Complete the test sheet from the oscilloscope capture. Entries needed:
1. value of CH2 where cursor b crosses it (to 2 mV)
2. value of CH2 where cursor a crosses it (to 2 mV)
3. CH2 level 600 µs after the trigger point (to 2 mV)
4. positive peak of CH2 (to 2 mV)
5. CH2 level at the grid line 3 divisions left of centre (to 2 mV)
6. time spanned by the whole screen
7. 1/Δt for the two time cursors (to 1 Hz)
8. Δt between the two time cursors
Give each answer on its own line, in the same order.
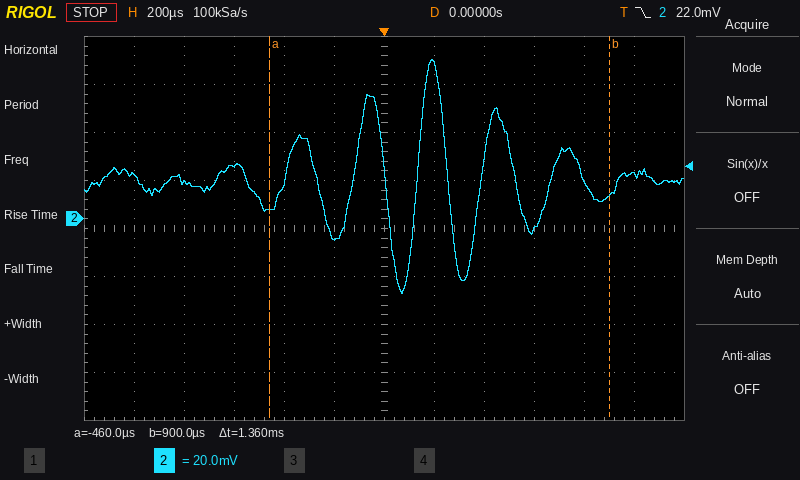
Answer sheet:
10 mV
4 mV
-4 mV
66 mV
22 mV
2.4 ms
735 Hz
1.36 ms
